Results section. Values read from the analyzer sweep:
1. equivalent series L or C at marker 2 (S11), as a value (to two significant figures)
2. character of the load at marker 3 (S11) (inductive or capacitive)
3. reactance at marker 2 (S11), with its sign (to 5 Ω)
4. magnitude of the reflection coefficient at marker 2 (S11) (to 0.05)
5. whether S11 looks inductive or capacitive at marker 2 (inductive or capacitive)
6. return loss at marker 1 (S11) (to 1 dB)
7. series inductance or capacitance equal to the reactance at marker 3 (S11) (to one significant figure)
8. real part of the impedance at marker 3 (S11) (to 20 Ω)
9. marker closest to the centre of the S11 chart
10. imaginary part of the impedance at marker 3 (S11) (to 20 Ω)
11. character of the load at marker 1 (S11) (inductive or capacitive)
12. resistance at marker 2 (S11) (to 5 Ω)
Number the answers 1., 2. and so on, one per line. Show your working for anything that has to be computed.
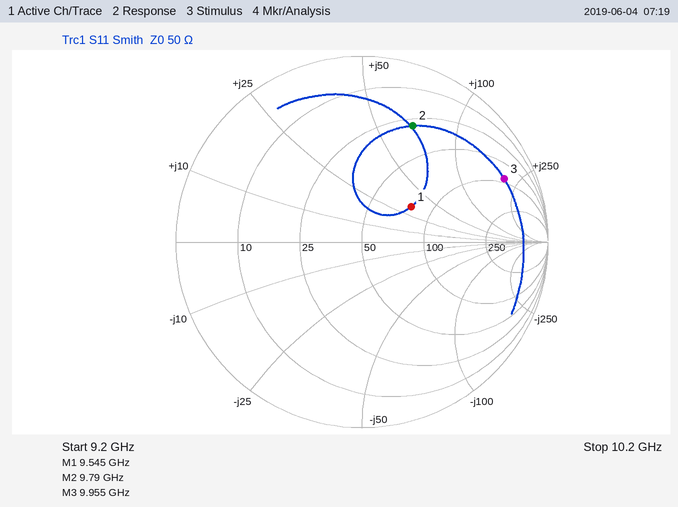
1. L = 70 Ω/(2π × 9.79 GHz) ≈ 1.1 nH
2. inductive
3. +70 Ω
4. 0.70
5. inductive
6. 10 dB
7. L = 200 Ω/(2π × 9.955 GHz) ≈ 3 nH
8. 80 Ω
9. marker 1
10. +200 Ω
11. inductive
12. 30 Ω
